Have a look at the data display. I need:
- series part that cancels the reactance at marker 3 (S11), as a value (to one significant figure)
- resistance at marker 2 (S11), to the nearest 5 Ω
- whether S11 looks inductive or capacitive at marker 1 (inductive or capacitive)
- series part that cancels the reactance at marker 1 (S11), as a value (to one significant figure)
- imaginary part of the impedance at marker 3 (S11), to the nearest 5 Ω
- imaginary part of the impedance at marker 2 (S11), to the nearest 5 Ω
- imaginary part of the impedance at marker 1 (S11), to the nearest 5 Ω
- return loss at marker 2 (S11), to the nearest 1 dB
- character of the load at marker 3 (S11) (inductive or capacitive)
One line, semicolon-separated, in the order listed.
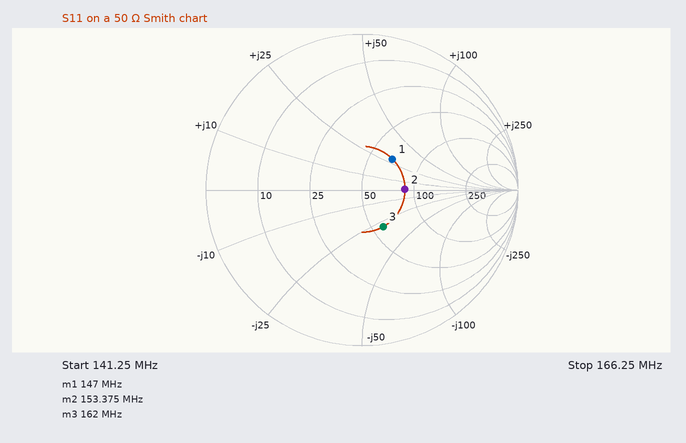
30 nH; 90 Ω; inductive; 40 pF; -30 Ω; 0 Ω; +30 Ω; 11 dB; capacitive
